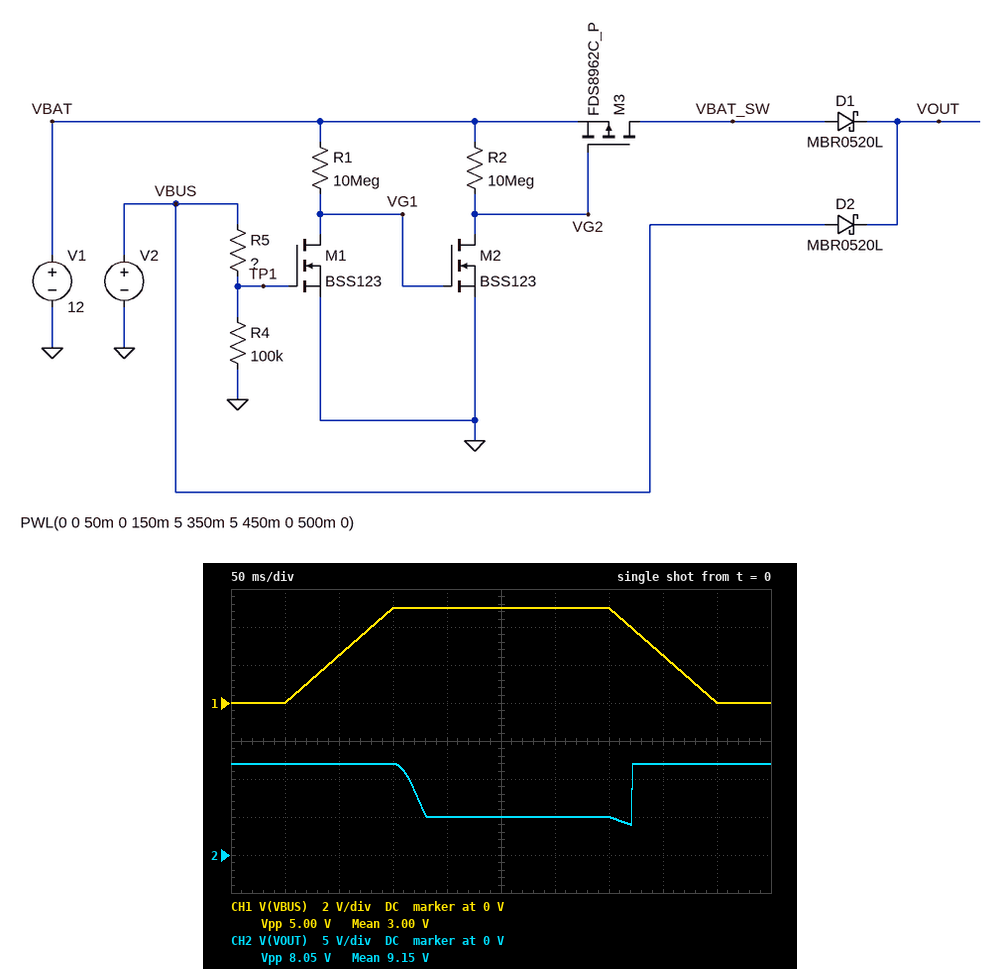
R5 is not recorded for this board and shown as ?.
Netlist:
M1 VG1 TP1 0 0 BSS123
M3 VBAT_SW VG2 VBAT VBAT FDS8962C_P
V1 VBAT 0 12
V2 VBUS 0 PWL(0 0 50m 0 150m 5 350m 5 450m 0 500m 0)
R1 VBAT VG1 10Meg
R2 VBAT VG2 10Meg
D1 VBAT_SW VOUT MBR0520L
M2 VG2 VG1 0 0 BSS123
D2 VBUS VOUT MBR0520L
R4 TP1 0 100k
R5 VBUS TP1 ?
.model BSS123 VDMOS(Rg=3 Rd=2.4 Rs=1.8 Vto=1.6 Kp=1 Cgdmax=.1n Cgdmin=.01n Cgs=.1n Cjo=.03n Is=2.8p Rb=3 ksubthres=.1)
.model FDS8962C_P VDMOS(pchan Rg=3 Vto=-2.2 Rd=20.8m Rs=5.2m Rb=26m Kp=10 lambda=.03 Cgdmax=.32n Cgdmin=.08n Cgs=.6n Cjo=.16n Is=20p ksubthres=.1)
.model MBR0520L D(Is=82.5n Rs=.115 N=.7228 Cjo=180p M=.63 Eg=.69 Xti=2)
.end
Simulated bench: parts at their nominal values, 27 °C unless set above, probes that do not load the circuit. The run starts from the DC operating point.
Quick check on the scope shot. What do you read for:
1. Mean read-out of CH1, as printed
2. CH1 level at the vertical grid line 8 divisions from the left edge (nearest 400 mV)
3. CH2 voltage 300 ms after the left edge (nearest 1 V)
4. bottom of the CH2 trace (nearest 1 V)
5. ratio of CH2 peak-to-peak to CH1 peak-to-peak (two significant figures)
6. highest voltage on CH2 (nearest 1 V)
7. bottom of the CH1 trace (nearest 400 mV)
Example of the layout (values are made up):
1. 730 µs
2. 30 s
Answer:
1. 3.00 V
2. 2.4 V
3. 5 V
4. 4 V
5. 1.6
6. 12 V
7. 0 V
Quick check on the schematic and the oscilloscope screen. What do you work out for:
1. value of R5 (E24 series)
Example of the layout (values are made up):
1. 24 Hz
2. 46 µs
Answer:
1. 240 kΩ
